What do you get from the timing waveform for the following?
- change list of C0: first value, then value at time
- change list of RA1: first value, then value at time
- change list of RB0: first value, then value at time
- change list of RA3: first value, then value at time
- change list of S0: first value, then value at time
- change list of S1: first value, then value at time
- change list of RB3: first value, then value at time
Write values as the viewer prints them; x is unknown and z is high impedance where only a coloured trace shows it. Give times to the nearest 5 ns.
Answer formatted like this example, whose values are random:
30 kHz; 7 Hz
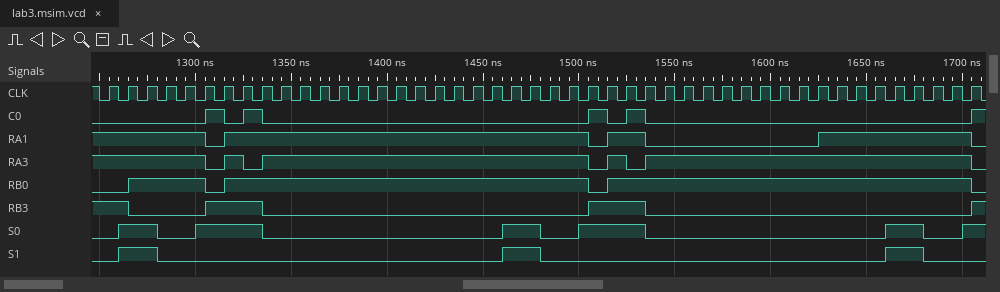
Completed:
0, 1 at 1305 ns, 0 at 1315 ns, 1 at 1325 ns, 0 at 1335 ns, 1 at 1505 ns, 0 at 1515 ns, 1 at 1525 ns, 0 at 1535 ns, 1 at 1705 ns; 1, 0 at 1305 ns, 1 at 1315 ns, 0 at 1505 ns, 1 at 1515 ns, 0 at 1535 ns, 1 at 1625 ns, 0 at 1705 ns; 0, 1 at 1265 ns, 0 at 1305 ns, 1 at 1315 ns, 0 at 1505 ns, 1 at 1515 ns, 0 at 1705 ns; 1, 0 at 1305 ns, 1 at 1315 ns, 0 at 1325 ns, 1 at 1335 ns, 0 at 1505 ns, 1 at 1515 ns, 0 at 1525 ns, 1 at 1535 ns, 0 at 1705 ns; 0, 1 at 1260 ns, 0 at 1280 ns, 1 at 1300 ns, 0 at 1335 ns, 1 at 1460 ns, 0 at 1480 ns, 1 at 1500 ns, 0 at 1535 ns, 1 at 1660 ns, 0 at 1680 ns, 1 at 1700 ns; 0, 1 at 1260 ns, 0 at 1280 ns, 1 at 1460 ns, 0 at 1480 ns, 1 at 1660 ns, 0 at 1680 ns; 1, 0 at 1265 ns, 1 at 1305 ns, 0 at 1335 ns, 1 at 1505 ns, 0 at 1535 ns, 1 at 1705 ns
